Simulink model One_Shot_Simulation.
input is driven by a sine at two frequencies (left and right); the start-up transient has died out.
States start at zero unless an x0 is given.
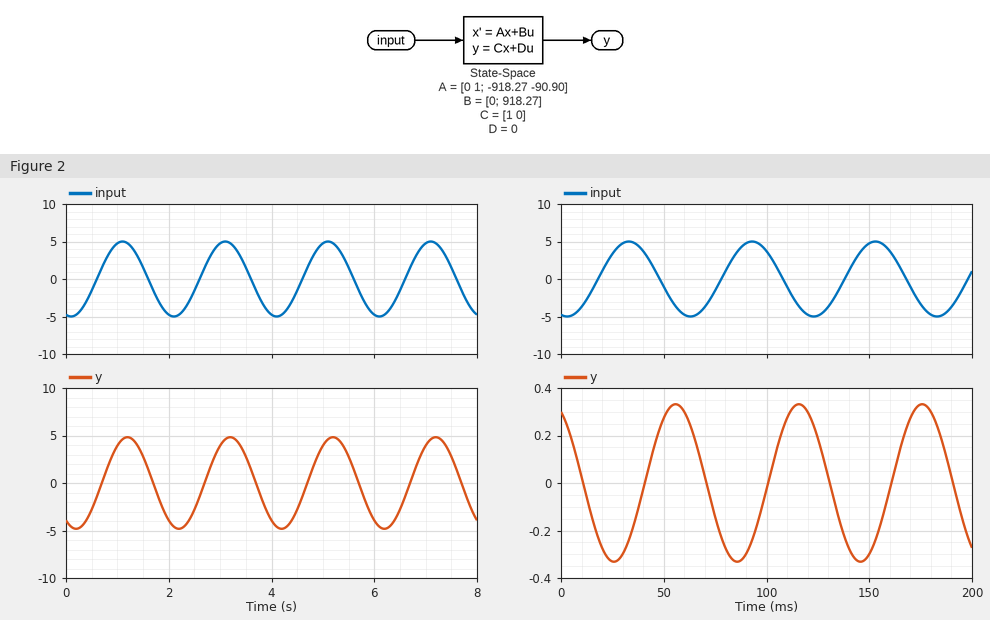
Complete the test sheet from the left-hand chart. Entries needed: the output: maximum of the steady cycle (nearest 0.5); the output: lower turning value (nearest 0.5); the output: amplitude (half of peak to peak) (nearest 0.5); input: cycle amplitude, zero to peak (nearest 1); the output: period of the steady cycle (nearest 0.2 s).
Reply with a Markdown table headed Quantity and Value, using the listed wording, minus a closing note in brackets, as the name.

| Quantity | Value |
|---|---|
| the output: maximum of the steady cycle | 5.0 |
| the output: lower turning value | -5.0 |
| the output: amplitude (half of peak to peak) | 5.0 |
| input: cycle amplitude, zero to peak | 5 |
| the output: period of the steady cycle | 2.0 s |
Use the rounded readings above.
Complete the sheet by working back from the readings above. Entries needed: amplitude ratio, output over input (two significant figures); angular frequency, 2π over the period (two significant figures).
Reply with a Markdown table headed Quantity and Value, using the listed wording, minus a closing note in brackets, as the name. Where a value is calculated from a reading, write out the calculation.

| Quantity | Value |
|---|---|
| amplitude ratio, output over input | 5 / 5 = 1.0 |
| angular frequency, 2π over the period | 2π / 2 = 3.1 rad/s |
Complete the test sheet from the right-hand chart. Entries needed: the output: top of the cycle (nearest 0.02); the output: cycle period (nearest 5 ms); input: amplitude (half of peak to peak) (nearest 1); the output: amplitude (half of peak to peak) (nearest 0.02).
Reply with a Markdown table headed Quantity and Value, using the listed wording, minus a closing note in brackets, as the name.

| Quantity | Value |
|---|---|
| the output: top of the cycle | 0.34 |
| the output: cycle period | 60 ms |
| input: amplitude (half of peak to peak) | 5 |
| the output: amplitude (half of peak to peak) | 0.34 |
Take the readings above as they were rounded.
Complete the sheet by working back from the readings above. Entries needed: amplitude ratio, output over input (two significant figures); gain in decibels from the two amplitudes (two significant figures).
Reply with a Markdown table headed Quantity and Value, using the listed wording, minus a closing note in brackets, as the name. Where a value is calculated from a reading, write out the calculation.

| Quantity | Value |
|---|---|
| amplitude ratio, output over input | 0.34 / 5 = 0.068 |
| gain in decibels from the two amplitudes | 20 log10(0.34 / 5) = -23 dB |
